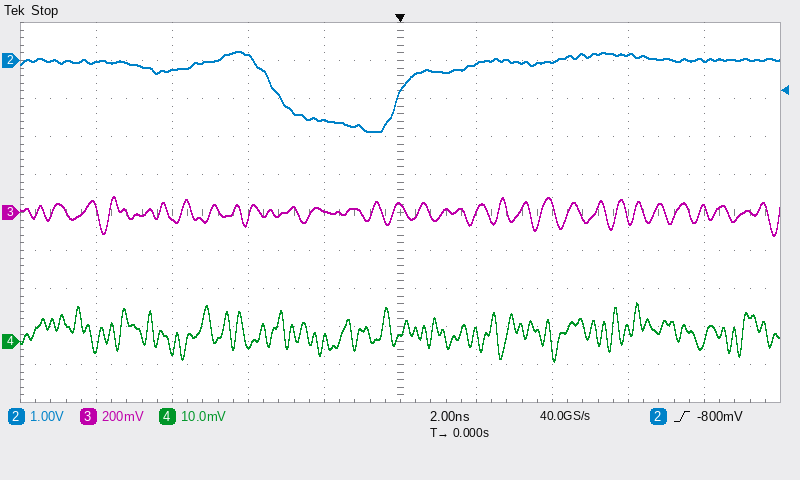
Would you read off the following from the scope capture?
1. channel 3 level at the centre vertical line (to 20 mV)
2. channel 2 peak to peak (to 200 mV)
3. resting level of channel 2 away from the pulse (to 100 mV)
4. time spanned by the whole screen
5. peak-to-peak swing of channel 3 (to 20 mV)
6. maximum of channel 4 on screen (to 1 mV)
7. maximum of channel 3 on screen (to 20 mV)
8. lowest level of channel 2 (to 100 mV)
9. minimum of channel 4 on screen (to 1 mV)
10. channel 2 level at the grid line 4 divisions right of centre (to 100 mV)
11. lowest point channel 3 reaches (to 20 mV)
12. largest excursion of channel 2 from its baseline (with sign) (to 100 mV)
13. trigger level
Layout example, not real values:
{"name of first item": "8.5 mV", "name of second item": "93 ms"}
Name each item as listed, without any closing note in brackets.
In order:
{"channel 3 level at the centre vertical line": "40 mV", "channel 2 peak to peak": "2.2 V", "resting level of channel 2 away from the pulse": "0.0 V", "time spanned by the whole screen": "20 ns", "peak-to-peak swing of channel 3": "200 mV", "maximum of channel 4 on screen": "10 mV", "maximum of channel 3 on screen": "80 mV", "lowest level of channel 2": "-1.9 V", "minimum of channel 4 on screen": "-5 mV", "channel 2 level at the grid line 4 divisions right of centre": "0.0 V", "lowest point channel 3 reaches": "-120 mV", "largest excursion of channel 2 from its baseline (with sign)": "-1.9 V", "trigger level": "-800 mV"}
